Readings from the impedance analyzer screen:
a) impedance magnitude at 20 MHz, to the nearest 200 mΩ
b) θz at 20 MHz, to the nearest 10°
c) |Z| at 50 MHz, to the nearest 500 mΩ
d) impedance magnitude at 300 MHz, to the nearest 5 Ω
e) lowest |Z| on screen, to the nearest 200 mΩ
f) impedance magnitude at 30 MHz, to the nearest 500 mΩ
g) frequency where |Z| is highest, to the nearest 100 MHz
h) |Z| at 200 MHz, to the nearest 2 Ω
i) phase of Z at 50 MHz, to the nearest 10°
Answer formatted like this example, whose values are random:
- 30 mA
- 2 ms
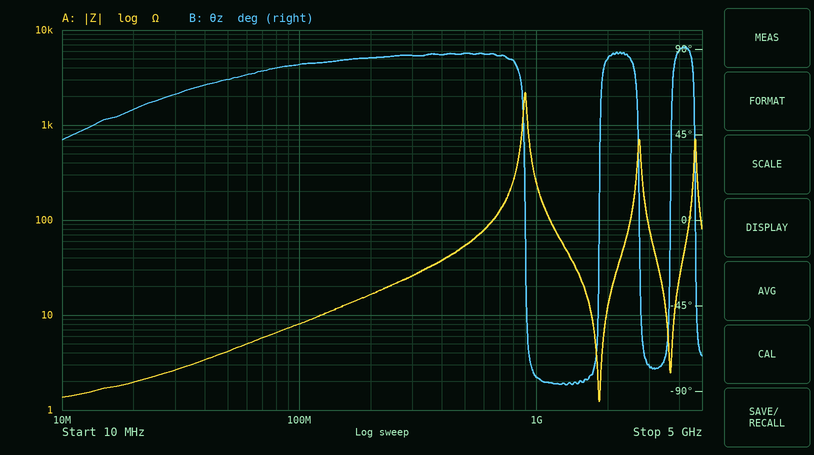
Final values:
- 2.0 Ω
- 60°
- 4.0 Ω
- 25 Ω
- 1.2 Ω
- 2.5 Ω
- 900 MHz
- 16 Ω
- 70°
